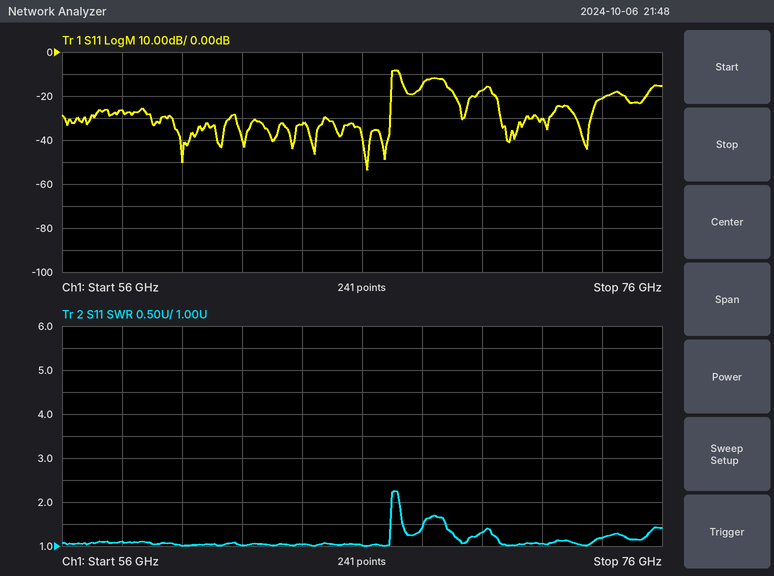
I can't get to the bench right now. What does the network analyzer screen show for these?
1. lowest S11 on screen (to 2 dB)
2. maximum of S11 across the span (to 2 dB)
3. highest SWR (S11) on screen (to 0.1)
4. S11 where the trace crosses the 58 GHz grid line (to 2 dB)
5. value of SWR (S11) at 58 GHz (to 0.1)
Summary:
-54 dB
-8 dB
2.3
-26 dB
1.1
